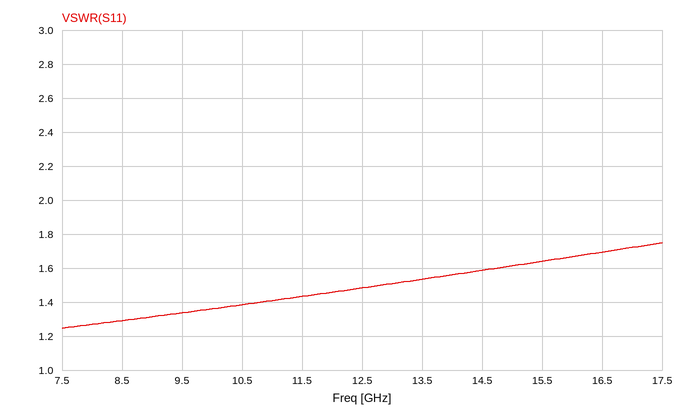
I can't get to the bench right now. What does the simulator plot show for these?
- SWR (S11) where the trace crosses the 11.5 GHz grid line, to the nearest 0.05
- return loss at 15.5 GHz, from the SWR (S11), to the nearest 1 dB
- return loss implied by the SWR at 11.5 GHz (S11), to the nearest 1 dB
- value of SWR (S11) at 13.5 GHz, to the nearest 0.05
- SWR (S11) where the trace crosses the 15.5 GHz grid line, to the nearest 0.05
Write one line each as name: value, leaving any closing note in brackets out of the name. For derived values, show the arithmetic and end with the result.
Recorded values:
SWR (S11) where the trace crosses the 11.5 GHz grid line, to the nearest 0.05: 1.45
return loss at 15.5 GHz, from the SWR (S11), to the nearest 1 dB: −20 log10((1.65 − 1)/(1.65 + 1)) ≈ 12 dB
return loss implied by the SWR at 11.5 GHz (S11), to the nearest 1 dB: −20 log10((1.45 − 1)/(1.45 + 1)) ≈ 15 dB
value of SWR (S11) at 13.5 GHz, to the nearest 0.05: 1.55
SWR (S11) where the trace crosses the 15.5 GHz grid line, to the nearest 0.05: 1.65
